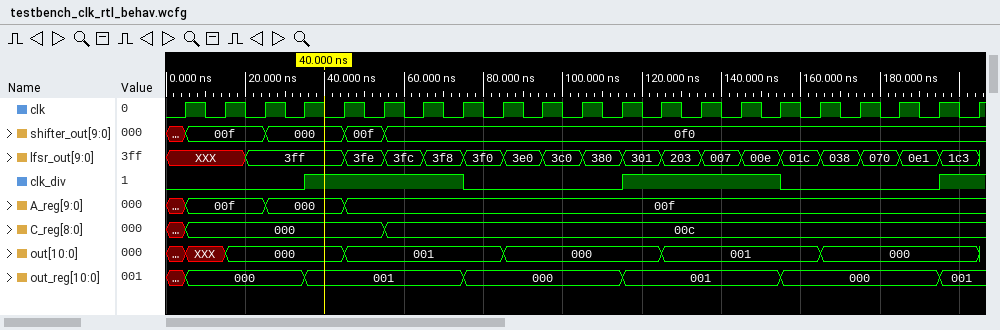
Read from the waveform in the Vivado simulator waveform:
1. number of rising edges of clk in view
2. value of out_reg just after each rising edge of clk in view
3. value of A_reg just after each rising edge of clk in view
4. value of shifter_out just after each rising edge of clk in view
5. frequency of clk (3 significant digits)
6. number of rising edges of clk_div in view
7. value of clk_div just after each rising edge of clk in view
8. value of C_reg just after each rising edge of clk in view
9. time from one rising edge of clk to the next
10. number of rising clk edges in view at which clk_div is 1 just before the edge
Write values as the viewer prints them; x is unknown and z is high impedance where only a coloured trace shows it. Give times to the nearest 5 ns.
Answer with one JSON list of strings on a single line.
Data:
["21", "000, 000, 000, 001, 001, 001, 001, 000, 000, 000, 000, 001, 001, 001, 001, 000, 000, 000, 000, 001, 001", "00f, 00f, 000, 000, 00f, 00f, 00f, 00f, 00f, 00f, 00f, 00f, 00f, 00f, 00f, 00f, 00f, 00f, 00f, 00f, 00f", "00f, 00f, 000, 000, 00f, 0f0, 0f0, 0f0, 0f0, 0f0, 0f0, 0f0, 0f0, 0f0, 0f0, 0f0, 0f0, 0f0, 0f0, 0f0, 0f0", "100 MHz", "3", "0 0 0 1 1 1 1 0 0 0 0 1 1 1 1 0 0 0 0 1 1", "000, 000, 000, 000, 000, 00c, 00c, 00c, 00c, 00c, 00c, 00c, 00c, 00c, 00c, 00c, 00c, 00c, 00c, 00c, 00c", "10 ns", "9"]
